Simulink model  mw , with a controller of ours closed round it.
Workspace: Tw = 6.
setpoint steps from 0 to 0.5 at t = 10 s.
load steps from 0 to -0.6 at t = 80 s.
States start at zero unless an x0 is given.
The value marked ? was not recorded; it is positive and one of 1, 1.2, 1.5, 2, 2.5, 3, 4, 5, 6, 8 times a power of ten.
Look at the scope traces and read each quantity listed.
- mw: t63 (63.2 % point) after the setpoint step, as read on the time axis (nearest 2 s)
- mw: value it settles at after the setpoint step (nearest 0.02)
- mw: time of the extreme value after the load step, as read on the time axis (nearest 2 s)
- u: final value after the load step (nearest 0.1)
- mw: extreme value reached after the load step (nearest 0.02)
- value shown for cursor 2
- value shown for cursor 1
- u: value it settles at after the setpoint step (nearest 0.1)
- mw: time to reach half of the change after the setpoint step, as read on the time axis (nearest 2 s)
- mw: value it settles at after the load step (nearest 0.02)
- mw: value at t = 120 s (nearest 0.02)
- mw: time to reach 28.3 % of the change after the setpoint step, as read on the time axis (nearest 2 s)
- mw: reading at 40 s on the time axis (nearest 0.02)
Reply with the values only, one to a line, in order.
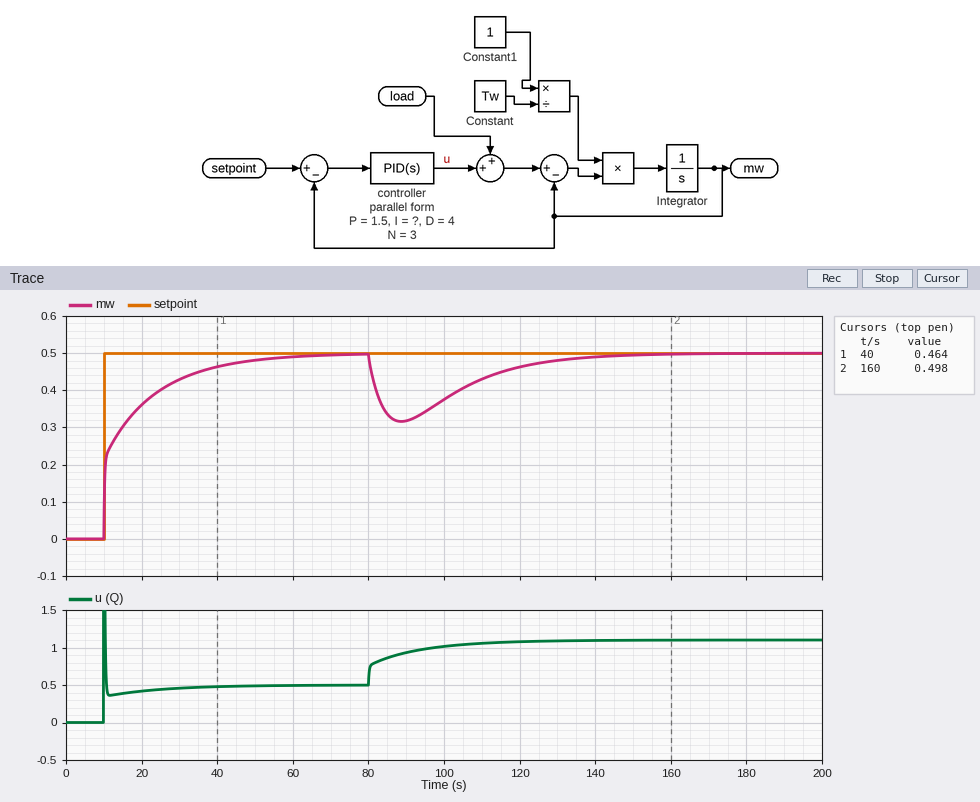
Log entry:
16 s
0.50
88 s
1.1
0.32
0.498
0.464
0.5
12 s
0.50
0.46
10 s
0.46
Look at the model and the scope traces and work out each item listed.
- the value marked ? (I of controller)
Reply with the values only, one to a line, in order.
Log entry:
0.12
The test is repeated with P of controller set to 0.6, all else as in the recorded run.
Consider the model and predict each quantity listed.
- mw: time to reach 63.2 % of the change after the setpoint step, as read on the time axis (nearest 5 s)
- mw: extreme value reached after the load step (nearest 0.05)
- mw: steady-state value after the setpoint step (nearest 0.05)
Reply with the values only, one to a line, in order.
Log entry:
20 s
0.25
0.50
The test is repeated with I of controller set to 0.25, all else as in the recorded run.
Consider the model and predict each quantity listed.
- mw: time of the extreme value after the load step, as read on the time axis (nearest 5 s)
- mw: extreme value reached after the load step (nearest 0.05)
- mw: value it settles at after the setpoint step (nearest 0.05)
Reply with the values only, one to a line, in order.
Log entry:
85 s
0.35
0.50
